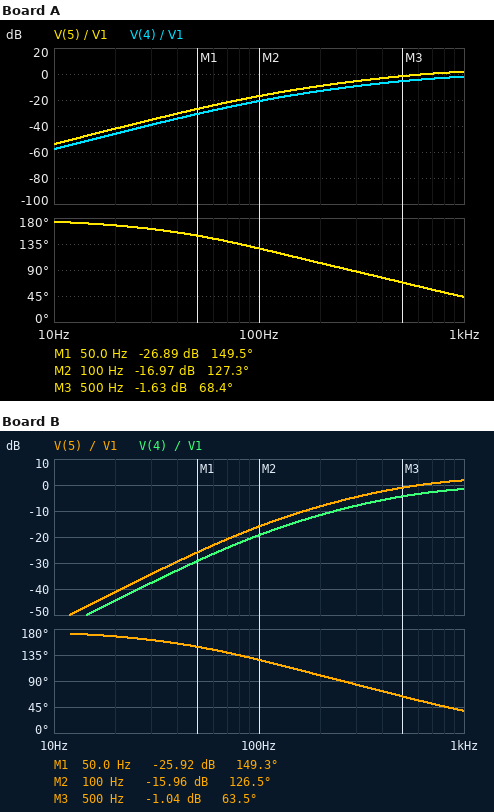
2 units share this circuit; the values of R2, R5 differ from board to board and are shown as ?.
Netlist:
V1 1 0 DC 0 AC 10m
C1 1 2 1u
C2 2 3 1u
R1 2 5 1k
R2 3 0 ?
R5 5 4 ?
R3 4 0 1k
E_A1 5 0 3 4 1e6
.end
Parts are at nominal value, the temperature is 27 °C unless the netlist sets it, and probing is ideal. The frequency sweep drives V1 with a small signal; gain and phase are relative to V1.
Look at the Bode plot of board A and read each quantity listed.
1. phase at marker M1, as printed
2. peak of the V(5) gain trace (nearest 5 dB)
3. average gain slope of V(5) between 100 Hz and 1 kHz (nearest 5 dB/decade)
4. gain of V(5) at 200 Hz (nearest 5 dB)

149.5 deg
0 dB
20 dB/decade
-10 dB
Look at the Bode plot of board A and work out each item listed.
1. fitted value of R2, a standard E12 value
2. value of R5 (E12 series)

330 Ω
560 Ω
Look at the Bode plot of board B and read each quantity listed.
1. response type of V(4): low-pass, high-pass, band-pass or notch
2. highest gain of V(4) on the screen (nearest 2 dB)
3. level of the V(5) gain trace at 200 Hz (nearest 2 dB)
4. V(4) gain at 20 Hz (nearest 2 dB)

high-pass
-2 dB
-8 dB
-44 dB
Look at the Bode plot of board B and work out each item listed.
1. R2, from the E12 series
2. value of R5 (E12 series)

390 Ω
470 Ω
